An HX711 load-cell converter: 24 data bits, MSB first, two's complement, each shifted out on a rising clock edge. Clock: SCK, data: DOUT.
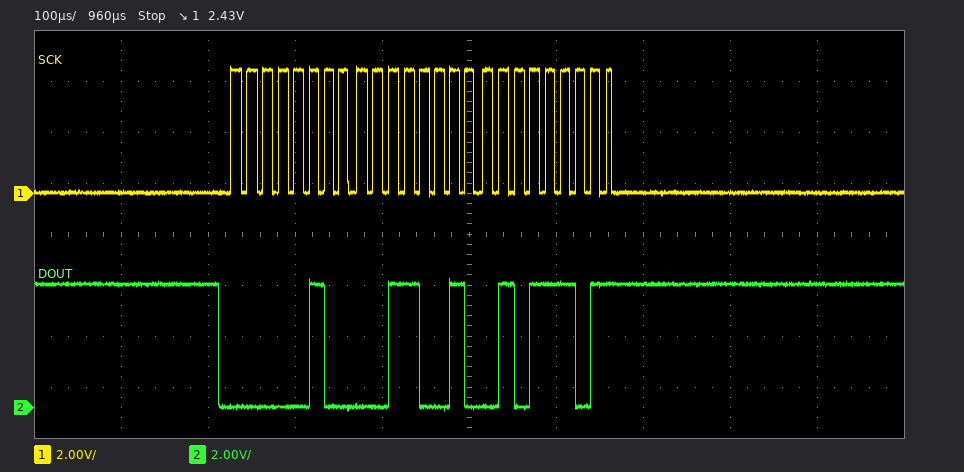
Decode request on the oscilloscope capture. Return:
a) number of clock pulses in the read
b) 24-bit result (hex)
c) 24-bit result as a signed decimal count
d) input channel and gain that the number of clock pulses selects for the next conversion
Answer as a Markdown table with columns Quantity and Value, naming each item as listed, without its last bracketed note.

| Quantity | Value |
|---|---|
| number of clock pulses in the read | 25 |
| 24-bit result | 0x04325D |
| 24-bit result as a signed decimal count | 275037 |
| input channel and gain that the number of clock pulses selects for the next conversion | channel A, gain 128 |
